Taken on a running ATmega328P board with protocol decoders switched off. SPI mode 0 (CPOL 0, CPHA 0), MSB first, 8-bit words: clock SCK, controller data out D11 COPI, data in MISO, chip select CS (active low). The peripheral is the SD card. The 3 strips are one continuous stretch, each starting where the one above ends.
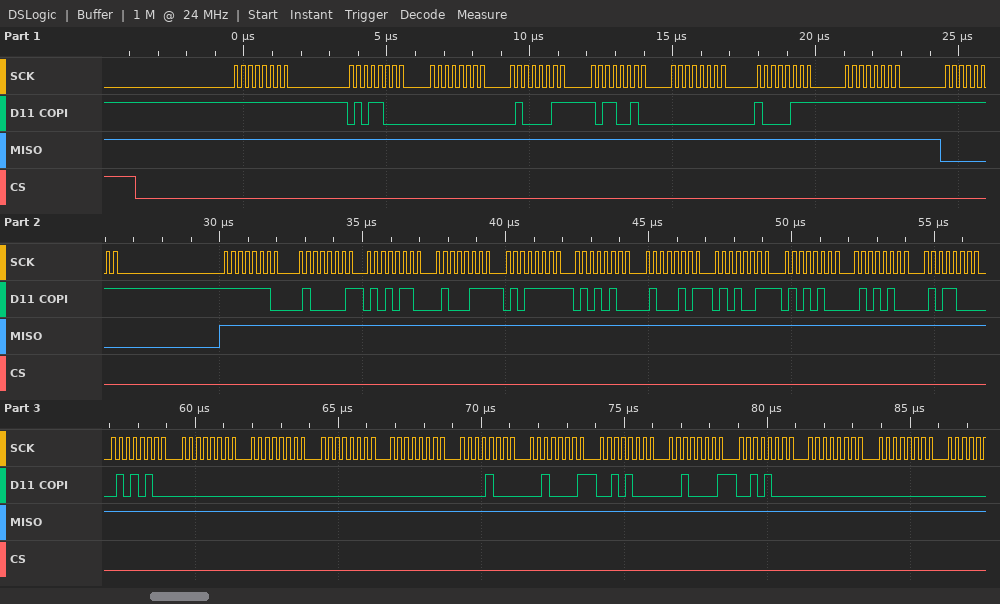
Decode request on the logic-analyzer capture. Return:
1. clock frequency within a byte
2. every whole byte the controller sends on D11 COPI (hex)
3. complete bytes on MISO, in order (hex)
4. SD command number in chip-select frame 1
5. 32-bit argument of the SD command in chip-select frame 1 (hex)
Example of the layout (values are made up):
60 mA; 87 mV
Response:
4 MHz; FF 58 00 43 B2 00 87 FF FF FE 41 56 47 5F 54 45 53 54 54 58 54 00 00 00 00 08 21 28 21 28 00 00; FF FF FF FF FF FF FF FF 00 FF FF FF FF FF FF FF FF FF FF FF FF FF FF FF FF FF FF FF FF FF FF FF; CMD24; 0x0043B200
